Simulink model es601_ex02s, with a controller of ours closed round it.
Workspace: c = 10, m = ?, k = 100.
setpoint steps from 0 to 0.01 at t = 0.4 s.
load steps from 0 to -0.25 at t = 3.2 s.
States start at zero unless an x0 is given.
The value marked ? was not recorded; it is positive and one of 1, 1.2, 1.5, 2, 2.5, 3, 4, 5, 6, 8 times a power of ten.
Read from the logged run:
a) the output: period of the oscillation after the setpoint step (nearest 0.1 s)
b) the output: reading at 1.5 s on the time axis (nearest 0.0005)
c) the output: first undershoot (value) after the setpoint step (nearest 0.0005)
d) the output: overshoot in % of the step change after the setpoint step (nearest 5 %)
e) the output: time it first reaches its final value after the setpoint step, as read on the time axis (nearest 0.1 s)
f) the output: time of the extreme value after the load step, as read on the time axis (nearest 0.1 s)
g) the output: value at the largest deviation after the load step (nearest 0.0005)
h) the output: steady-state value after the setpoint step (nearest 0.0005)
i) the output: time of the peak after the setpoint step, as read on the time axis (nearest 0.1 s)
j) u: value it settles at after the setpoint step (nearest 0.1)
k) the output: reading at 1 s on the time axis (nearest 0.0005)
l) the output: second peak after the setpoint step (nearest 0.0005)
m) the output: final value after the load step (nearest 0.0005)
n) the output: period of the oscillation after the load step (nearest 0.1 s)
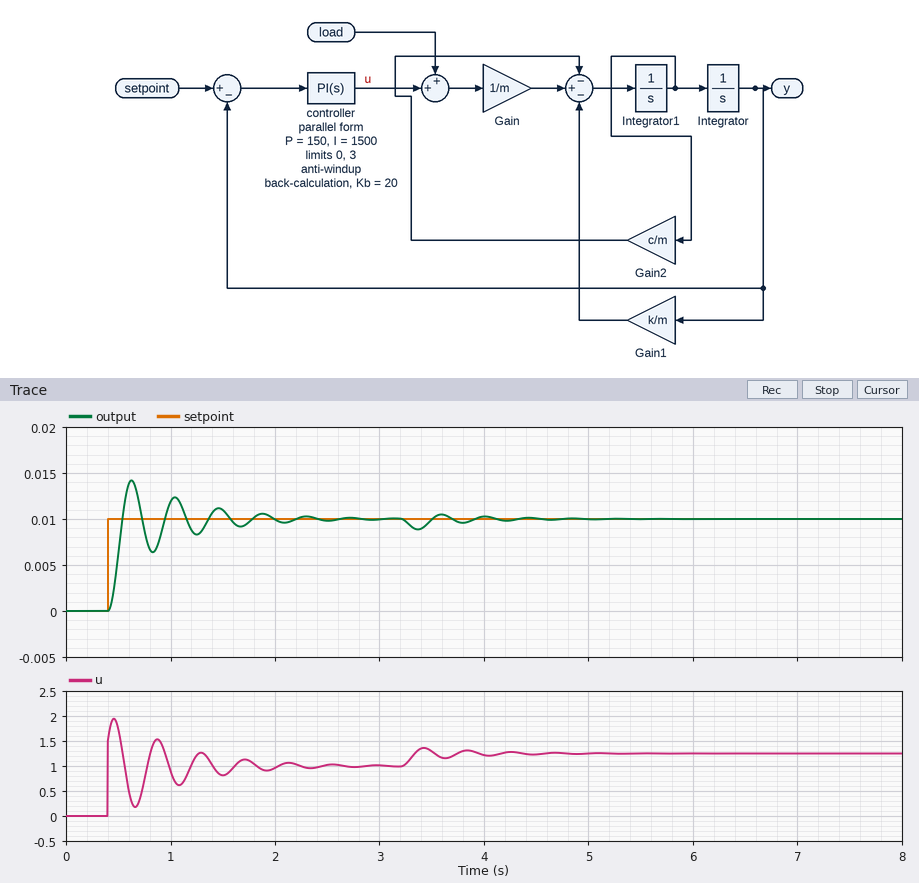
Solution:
0.4 s
0.0110
0.0065
40 %
0.5 s
3.4 s
0.0090
0.0100
0.6 s
1.0
0.0120
0.0125
0.0100
0.4 s
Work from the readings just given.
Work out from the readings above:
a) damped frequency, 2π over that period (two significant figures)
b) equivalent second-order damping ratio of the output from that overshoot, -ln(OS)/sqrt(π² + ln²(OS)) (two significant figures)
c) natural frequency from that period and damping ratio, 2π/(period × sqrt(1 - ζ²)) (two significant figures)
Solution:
16 rad/s
0.28
16 rad/s
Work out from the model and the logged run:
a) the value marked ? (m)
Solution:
1
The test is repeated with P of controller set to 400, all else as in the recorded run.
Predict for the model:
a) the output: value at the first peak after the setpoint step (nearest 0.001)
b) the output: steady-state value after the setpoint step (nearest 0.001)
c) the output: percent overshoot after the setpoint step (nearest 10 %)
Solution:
0.013
0.010
30 %
